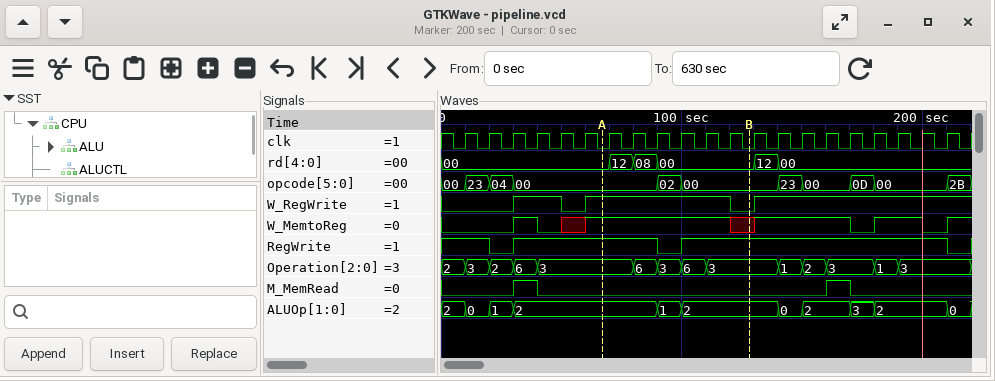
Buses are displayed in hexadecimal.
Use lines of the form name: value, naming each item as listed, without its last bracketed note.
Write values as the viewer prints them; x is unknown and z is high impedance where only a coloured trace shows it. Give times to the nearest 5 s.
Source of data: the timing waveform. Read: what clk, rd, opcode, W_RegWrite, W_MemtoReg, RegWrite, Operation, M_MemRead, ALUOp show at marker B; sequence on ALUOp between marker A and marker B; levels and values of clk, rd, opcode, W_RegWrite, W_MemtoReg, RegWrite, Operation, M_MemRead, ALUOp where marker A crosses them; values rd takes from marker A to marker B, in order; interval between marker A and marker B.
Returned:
what clk, rd, opcode, W_RegWrite, W_MemtoReg, RegWrite, Operation, M_MemRead, ALUOp show at marker B: clk=0, rd=00, opcode=00, W_RegWrite=0, W_MemtoReg=x, RegWrite=1, Operation=3, M_MemRead=0, ALUOp=2
sequence on ALUOp between marker A and marker B: 2, 1, 2
levels and values of clk, rd, opcode, W_RegWrite, W_MemtoReg, RegWrite, Operation, M_MemRead, ALUOp where marker A crosses them: clk=0, rd=00, opcode=00, W_RegWrite=1, W_MemtoReg=1, RegWrite=1, Operation=3, M_MemRead=0, ALUOp=2
values rd takes from marker A to marker B, in order: 00, 12, 08, 00
interval between marker A and marker B: 60 s
